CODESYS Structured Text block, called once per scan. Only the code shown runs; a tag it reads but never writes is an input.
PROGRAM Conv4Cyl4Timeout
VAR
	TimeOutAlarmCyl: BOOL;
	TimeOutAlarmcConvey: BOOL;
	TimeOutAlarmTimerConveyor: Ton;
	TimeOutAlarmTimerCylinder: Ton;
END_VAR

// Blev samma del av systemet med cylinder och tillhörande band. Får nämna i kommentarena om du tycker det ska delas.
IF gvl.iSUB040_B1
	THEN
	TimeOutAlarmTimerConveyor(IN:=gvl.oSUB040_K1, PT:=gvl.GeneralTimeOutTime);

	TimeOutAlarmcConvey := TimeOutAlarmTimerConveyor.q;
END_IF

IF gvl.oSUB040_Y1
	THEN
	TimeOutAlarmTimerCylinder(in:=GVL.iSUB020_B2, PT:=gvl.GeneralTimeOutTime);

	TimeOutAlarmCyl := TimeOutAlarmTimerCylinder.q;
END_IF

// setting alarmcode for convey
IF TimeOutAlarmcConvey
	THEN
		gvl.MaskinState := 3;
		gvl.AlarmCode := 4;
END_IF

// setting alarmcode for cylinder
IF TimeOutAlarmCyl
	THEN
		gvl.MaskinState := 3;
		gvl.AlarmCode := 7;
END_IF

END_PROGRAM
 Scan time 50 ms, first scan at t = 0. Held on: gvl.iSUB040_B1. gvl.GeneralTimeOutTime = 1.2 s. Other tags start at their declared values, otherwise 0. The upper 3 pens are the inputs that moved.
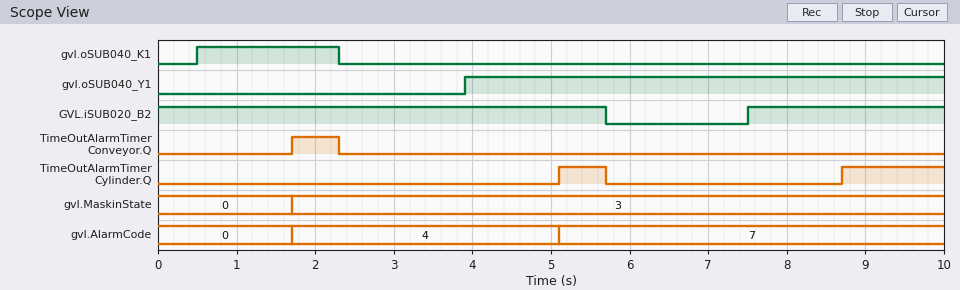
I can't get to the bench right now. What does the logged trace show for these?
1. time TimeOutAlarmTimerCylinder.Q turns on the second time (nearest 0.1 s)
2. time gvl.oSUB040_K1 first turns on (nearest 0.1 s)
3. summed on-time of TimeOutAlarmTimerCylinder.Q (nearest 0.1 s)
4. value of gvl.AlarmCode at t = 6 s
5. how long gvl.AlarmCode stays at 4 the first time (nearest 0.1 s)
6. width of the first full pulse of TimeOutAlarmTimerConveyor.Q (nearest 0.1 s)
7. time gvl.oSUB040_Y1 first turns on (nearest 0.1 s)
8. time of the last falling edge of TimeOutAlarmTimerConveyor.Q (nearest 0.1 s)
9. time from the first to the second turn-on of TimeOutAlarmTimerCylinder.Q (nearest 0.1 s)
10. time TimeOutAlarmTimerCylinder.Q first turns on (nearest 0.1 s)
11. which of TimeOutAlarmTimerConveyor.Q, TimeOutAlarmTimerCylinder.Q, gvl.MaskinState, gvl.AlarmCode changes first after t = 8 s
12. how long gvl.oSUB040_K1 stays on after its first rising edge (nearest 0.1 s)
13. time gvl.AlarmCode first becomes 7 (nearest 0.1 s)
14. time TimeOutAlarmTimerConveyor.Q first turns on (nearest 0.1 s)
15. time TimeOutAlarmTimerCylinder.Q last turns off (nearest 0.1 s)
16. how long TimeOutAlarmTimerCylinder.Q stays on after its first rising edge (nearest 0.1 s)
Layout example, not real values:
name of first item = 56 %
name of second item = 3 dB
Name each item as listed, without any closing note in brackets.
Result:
time TimeOutAlarmTimerCylinder.Q turns on the second time = 8.7 s
time gvl.oSUB040_K1 first turns on = 0.5 s
summed on-time of TimeOutAlarmTimerCylinder.Q = 1.9 s
value of gvl.AlarmCode at t = 6 s = 7
how long gvl.AlarmCode stays at 4 the first time = 3.4 s
width of the first full pulse of TimeOutAlarmTimerConveyor.Q = 0.6 s
time gvl.oSUB040_Y1 first turns on = 3.9 s
time of the last falling edge of TimeOutAlarmTimerConveyor.Q = 2.3 s
time from the first to the second turn-on of TimeOutAlarmTimerCylinder.Q = 3.6 s
time TimeOutAlarmTimerCylinder.Q first turns on = 5.1 s
which of TimeOutAlarmTimerConveyor.Q, TimeOutAlarmTimerCylinder.Q, gvl.MaskinState, gvl.AlarmCode changes first after t = 8 s = TimeOutAlarmTimerCylinder.Q
how long gvl.oSUB040_K1 stays on after its first rising edge = 1.8 s
time gvl.AlarmCode first becomes 7 = 5.1 s
time TimeOutAlarmTimerConveyor.Q first turns on = 1.7 s
time TimeOutAlarmTimerCylinder.Q last turns off = 5.7 s
how long TimeOutAlarmTimerCylinder.Q stays on after its first rising edge = 0.6 s
